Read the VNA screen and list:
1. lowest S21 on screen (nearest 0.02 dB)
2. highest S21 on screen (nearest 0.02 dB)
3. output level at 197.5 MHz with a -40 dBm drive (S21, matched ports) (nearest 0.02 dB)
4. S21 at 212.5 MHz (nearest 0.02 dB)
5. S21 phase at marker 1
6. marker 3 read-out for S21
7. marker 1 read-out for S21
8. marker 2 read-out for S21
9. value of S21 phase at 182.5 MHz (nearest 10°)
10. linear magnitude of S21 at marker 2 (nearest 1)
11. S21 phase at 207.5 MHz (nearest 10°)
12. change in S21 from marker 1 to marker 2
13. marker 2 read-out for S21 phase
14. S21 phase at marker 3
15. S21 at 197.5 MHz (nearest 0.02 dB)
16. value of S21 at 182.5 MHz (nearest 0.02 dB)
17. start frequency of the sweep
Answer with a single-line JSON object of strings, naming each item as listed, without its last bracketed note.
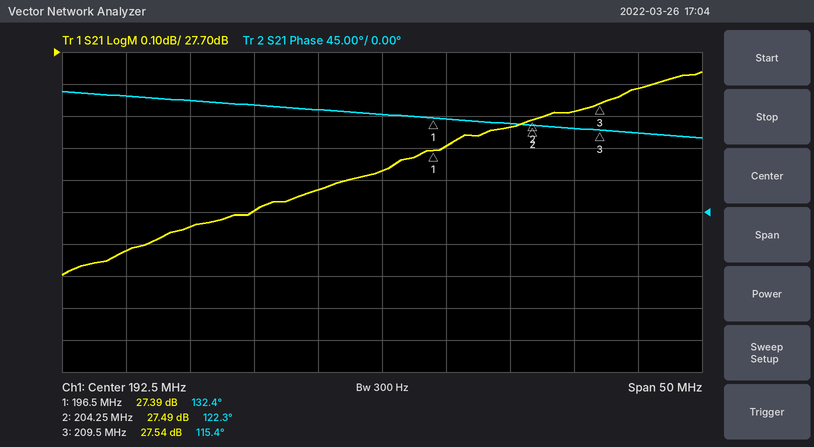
{"lowest S21 on screen": "27.00 dB", "highest S21 on screen": "27.64 dB", "output level at 197.5 MHz with a -40 dBm drive (S21, matched ports)": "-12.60 dBm", "S21 at 212.5 MHz": "27.58 dB", "S21 phase at marker 1": "132.4°", "marker 3 read-out for S21": "27.54 dB", "marker 1 read-out for S21": "27.39 dB", "marker 2 read-out for S21": "27.49 dB", "value of S21 phase at 182.5 MHz": "150°", "linear magnitude of S21 at marker 2": "24", "S21 phase at 207.5 MHz": "120°", "change in S21 from marker 1 to marker 2": "0.10 dB", "marker 2 read-out for S21 phase": "122.3°", "S21 phase at marker 3": "115.4°", "S21 at 197.5 MHz": "27.40 dB", "value of S21 at 182.5 MHz": "27.20 dB", "start frequency of the sweep": "167.5 MHz"}
